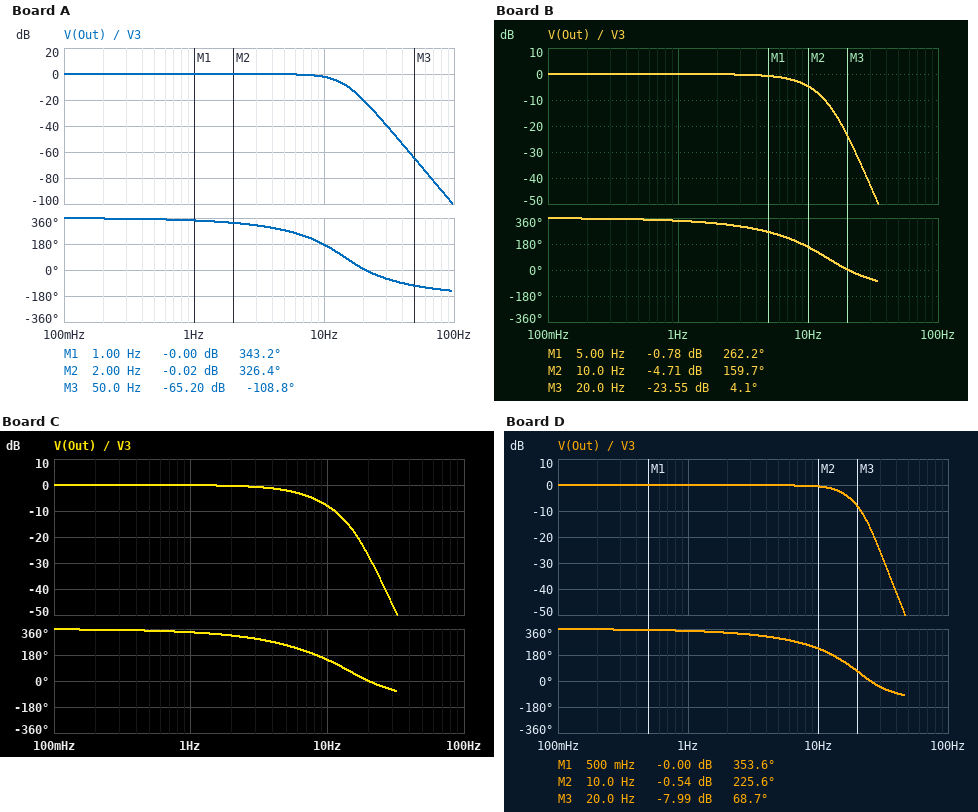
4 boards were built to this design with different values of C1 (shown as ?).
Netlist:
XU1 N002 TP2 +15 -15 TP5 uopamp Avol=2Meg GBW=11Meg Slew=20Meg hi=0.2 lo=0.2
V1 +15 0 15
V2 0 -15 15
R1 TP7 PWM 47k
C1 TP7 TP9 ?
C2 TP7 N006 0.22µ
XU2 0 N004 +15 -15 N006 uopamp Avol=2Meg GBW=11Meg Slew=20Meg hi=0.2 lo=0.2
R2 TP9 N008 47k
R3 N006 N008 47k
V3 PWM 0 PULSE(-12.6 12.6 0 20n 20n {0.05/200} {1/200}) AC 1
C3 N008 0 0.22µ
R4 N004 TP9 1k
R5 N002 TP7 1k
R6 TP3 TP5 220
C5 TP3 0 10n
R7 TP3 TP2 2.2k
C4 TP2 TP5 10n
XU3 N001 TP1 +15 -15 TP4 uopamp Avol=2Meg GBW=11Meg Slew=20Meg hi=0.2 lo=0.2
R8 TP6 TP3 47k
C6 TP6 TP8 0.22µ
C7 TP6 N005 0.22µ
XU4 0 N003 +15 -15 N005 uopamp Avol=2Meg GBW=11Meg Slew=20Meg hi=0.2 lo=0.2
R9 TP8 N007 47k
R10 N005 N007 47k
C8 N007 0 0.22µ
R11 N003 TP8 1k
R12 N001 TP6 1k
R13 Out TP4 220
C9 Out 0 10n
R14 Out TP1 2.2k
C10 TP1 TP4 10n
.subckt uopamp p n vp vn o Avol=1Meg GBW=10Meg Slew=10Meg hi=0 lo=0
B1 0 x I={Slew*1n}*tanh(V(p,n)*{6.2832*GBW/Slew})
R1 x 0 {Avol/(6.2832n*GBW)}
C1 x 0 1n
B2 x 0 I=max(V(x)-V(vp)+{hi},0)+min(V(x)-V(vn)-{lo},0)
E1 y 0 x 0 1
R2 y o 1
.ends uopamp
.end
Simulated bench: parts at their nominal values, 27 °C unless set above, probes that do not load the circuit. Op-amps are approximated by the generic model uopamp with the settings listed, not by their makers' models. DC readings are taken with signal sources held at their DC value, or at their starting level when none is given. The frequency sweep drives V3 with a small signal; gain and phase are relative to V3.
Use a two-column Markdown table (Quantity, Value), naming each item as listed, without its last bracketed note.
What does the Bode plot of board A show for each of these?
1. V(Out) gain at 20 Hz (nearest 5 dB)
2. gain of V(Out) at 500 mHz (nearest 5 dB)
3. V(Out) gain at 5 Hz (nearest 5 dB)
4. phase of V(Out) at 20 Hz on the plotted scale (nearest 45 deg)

| Quantity | Value |
|---|---|
| V(Out) gain at 20 Hz | -20 dB |
| gain of V(Out) at 500 mHz | 0 dB |
| V(Out) gain at 5 Hz | 0 dB |
| phase of V(Out) at 20 Hz on the plotted scale | 0 deg |
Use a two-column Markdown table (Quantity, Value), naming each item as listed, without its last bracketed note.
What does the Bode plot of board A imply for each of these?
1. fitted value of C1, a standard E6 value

| Quantity | Value |
|---|---|
| fitted value of C1, a standard E6 value | 330 nF |
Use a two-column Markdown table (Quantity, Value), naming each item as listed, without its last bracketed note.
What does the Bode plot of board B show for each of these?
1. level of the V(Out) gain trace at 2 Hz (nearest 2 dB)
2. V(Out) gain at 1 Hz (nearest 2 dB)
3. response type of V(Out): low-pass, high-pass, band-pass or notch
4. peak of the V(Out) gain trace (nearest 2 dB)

| Quantity | Value |
|---|---|
| level of the V(Out) gain trace at 2 Hz | 0 dB |
| V(Out) gain at 1 Hz | 0 dB |
| response type of V(Out): low-pass, high-pass, band-pass or notch | low-pass |
| peak of the V(Out) gain trace | 0 dB |
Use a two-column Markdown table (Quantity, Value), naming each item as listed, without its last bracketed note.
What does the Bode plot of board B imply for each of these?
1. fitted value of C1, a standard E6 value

| Quantity | Value |
|---|---|
| fitted value of C1, a standard E6 value | 470 nF |
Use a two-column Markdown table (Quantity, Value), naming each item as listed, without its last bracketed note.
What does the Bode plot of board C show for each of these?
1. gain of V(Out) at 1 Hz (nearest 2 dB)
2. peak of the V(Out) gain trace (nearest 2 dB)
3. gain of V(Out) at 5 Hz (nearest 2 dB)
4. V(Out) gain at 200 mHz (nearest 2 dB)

| Quantity | Value |
|---|---|
| gain of V(Out) at 1 Hz | 0 dB |
| peak of the V(Out) gain trace | 0 dB |
| gain of V(Out) at 5 Hz | -2 dB |
| V(Out) gain at 200 mHz | 0 dB |
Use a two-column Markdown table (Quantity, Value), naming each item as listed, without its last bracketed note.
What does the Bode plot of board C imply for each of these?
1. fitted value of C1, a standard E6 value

| Quantity | Value |
|---|---|
| fitted value of C1, a standard E6 value | 680 nF |
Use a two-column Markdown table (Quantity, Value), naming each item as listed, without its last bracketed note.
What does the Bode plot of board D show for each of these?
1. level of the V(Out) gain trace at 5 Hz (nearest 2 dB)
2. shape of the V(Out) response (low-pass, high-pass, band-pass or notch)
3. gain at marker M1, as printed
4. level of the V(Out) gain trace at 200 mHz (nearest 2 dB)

| Quantity | Value |
|---|---|
| level of the V(Out) gain trace at 5 Hz | 0 dB |
| shape of the V(Out) response | low-pass |
| gain at marker M1, as printed | -0.00 dB |
| level of the V(Out) gain trace at 200 mHz | 0 dB |
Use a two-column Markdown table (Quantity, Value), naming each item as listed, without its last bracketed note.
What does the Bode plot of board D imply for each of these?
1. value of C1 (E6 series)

| Quantity | Value |
|---|---|
| value of C1 | 100 nF |
